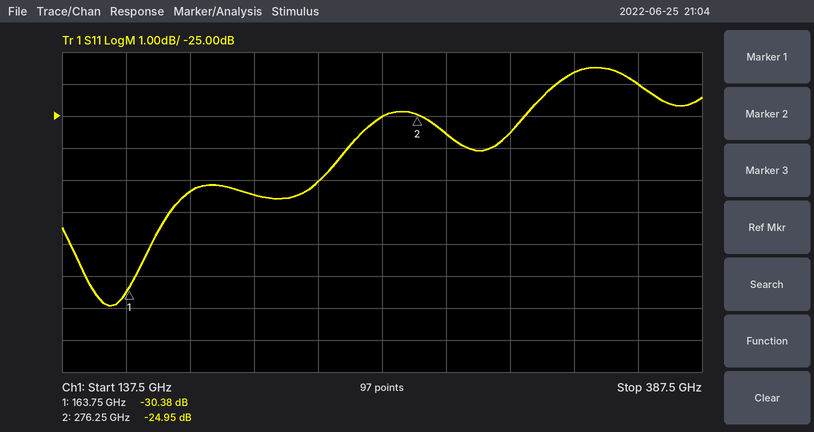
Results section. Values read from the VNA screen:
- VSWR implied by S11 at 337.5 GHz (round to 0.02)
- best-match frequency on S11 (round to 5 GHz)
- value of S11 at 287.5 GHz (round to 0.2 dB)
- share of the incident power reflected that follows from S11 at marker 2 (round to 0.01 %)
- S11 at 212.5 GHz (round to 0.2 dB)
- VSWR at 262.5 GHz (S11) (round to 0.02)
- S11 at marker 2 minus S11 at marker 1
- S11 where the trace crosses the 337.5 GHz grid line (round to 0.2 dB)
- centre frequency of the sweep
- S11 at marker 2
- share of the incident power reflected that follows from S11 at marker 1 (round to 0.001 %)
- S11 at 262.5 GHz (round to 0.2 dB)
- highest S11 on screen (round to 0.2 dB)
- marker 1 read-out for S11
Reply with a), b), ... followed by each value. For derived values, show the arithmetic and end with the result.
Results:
a) |Γ| = 10^(-23.6/20) = 0.0661; VSWR = (1 + 0.0661)/(1 − 0.0661) ≈ 1.14
b) 155 GHz
c) -25.6 dB
d) 10^(-24.95/10) ≈ 0.32 %
e) -27.4 dB
f) |Γ| = 10^(-25/20) = 0.0562; VSWR = (1 + 0.0562)/(1 − 0.0562) ≈ 1.12
g) -24.95 − (-30.38) = 5.43 dB
h) -23.6 dB
i) 262.5 GHz
j) -24.95 dB
k) 10^(-30.38/10) ≈ 0.092 %
l) -25.0 dB
m) -23.4 dB
n) -30.38 dB
